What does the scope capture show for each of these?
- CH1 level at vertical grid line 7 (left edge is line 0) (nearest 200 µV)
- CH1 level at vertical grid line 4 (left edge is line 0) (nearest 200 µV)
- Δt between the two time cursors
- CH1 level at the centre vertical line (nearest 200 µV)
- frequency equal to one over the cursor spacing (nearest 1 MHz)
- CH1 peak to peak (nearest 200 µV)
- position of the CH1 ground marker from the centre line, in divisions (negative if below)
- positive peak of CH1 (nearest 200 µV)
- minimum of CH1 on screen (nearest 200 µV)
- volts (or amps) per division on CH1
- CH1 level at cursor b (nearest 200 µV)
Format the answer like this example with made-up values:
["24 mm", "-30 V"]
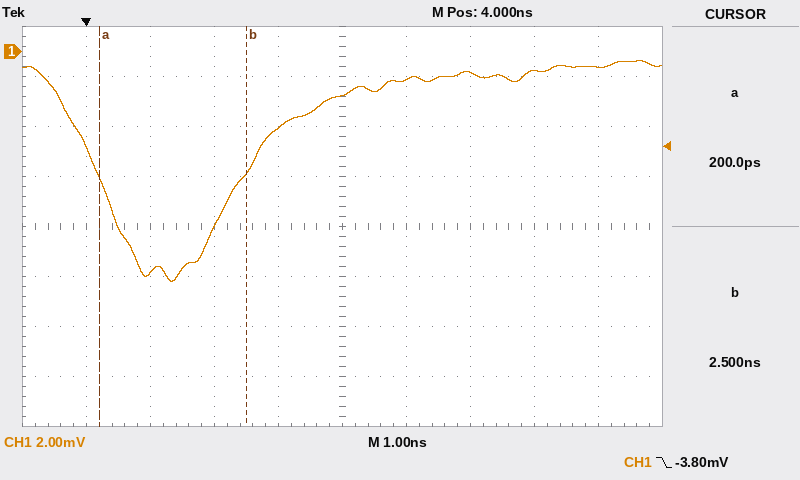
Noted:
["-800 µV", "-3.0 mV", "2.3 ns", "-1.8 mV", "435 MHz", "8.8 mV", "+3.5 div", "-400 µV", "-9.2 mV", "2 mV", "-4.8 mV"]
